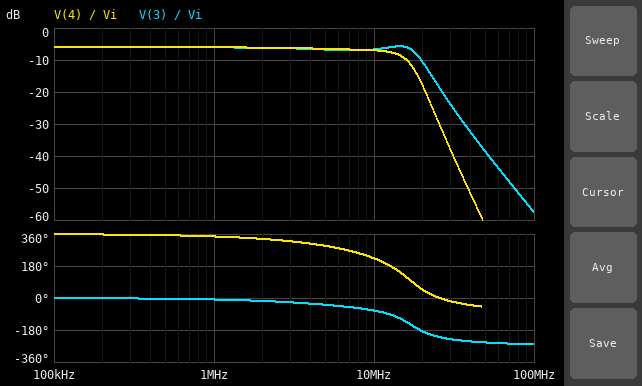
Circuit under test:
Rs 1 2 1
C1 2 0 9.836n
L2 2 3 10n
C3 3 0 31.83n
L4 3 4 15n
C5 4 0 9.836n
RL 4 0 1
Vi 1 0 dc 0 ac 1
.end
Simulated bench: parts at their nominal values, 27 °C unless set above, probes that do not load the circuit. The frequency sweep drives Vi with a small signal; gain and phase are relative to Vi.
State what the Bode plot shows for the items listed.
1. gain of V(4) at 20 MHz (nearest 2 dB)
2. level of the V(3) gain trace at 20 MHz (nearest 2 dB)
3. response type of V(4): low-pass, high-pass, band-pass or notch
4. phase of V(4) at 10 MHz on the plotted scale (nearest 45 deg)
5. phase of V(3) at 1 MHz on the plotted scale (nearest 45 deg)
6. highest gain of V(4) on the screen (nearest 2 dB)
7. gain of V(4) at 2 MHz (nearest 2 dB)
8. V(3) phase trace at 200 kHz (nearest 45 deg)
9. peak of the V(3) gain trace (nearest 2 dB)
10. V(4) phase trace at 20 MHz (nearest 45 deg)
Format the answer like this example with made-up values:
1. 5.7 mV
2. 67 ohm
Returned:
1. -18 dB
2. -10 dB
3. low-pass
4. 225 deg
5. 0 deg
6. -6 dB
7. -6 dB
8. 0 deg
9. -6 dB
10. 45 deg
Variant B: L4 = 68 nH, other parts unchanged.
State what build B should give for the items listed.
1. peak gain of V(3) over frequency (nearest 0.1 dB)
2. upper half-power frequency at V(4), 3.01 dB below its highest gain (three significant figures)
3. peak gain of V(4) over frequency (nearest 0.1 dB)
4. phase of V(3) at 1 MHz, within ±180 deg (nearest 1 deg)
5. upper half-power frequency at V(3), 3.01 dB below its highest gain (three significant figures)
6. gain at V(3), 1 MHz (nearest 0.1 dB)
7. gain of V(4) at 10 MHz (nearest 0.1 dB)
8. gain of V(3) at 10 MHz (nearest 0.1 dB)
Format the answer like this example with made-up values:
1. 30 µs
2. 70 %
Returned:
1. -2.6 dB
2. 4.84 MHz
3. -6.0 dB
4. 0 deg
5. 12.9 MHz
6. -5.5 dB
7. -17.9 dB
8. -4.7 dB
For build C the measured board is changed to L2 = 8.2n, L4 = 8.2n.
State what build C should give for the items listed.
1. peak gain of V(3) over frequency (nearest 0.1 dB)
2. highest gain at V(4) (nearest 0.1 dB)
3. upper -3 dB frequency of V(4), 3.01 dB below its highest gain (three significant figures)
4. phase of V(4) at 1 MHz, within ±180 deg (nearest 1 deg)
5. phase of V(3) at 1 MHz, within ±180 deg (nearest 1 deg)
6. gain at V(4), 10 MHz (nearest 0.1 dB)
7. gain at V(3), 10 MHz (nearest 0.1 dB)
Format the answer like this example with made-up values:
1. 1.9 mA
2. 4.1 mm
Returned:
1. -6.0 dB
2. -6.0 dB
3. 20.4 MHz
4. -12 deg
5. -9 deg
6. -7.5 dB
7. -8.9 dB
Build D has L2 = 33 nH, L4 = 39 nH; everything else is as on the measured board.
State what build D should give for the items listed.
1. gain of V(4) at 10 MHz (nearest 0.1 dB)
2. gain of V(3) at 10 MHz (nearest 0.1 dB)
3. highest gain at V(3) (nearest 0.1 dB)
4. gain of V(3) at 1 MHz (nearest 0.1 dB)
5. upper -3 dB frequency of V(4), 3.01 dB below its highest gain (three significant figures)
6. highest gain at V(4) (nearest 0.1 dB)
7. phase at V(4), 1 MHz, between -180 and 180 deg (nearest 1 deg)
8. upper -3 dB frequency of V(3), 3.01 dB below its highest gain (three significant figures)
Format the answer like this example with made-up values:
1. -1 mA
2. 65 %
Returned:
1. -15.3 dB
2. -7.4 dB
3. -1.9 dB
4. -5.9 dB
5. 8.19 MHz
6. -6.0 dB
7. -22 deg
8. 9.07 MHz
